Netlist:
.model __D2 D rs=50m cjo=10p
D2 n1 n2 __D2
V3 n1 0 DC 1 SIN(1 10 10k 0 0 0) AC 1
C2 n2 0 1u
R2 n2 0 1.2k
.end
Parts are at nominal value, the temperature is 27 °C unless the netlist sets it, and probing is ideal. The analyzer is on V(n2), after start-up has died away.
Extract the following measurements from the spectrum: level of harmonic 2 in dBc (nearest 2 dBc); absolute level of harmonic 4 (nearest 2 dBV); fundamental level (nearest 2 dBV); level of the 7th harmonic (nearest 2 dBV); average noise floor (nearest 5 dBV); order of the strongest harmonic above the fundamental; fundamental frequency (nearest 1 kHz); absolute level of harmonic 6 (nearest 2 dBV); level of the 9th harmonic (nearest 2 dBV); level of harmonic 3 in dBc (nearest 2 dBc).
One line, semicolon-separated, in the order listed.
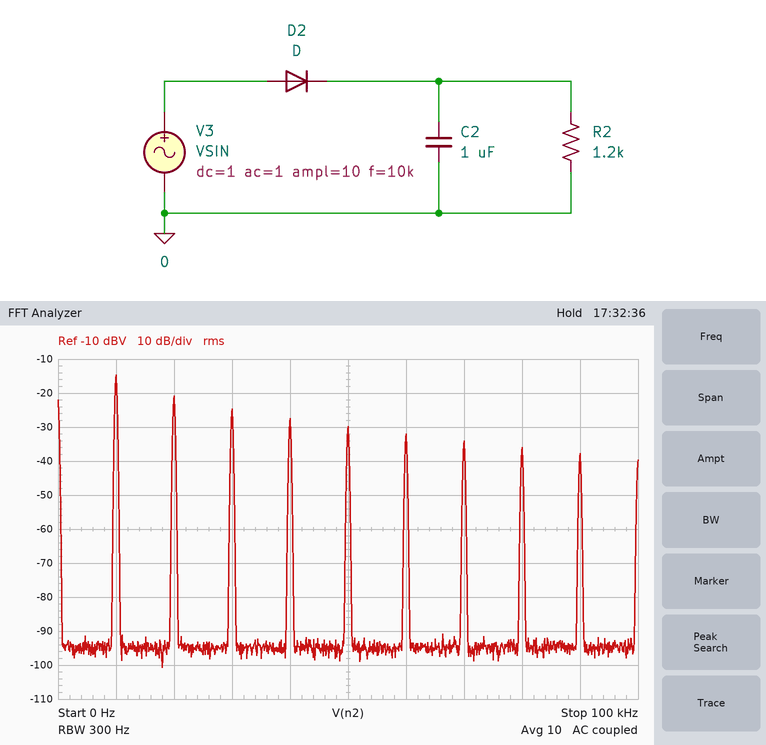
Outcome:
-6 dBc; -28 dBV; -14 dBV; -34 dBV; -95 dBV; 2; 10 kHz; -32 dBV; -38 dBV; -10 dBc
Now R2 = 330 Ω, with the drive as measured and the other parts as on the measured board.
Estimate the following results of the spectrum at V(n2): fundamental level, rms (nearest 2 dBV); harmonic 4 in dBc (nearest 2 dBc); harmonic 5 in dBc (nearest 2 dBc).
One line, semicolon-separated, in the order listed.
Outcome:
-4 dBV; -14 dBc; -18 dBc
